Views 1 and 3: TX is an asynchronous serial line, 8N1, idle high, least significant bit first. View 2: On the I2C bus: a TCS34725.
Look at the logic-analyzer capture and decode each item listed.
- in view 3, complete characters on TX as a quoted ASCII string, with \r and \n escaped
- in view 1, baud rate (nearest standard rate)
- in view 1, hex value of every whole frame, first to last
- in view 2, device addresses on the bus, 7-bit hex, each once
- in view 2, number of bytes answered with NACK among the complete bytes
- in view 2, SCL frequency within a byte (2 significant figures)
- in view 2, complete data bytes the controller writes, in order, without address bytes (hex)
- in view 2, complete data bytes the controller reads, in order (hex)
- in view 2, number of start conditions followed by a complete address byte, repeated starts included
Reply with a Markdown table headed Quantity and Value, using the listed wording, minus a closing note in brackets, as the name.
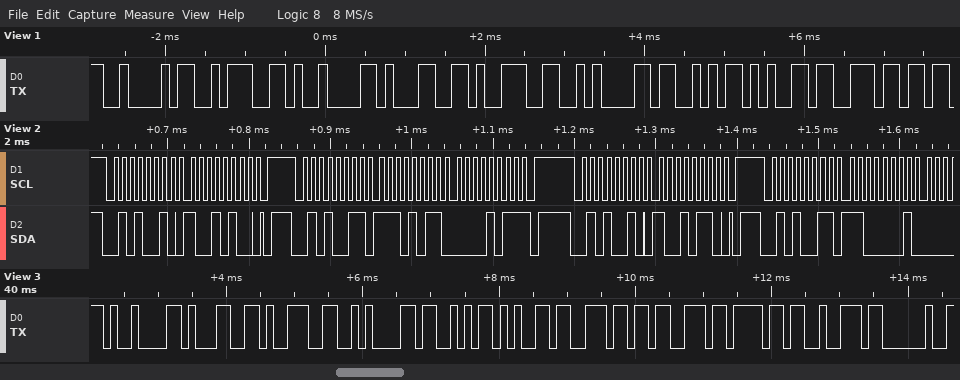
| Quantity | Value |
|---|---|
| in view 3, complete characters on TX as a quoted ASCII string, with \r and \n escaped | "\t19\nSensor " |
| in view 1, baud rate | 9600 baud |
| in view 1, hex value of every whole frame, first to last | 42 3A 09 31 39 0A 53 65 6E |
| in view 2, device addresses on the bus, 7-bit hex, each once | 0x29 |
| in view 2, number of bytes answered with NACK among the complete bytes | 1 |
| in view 2, SCL frequency within a byte | 100 kHz |
| in view 2, complete data bytes the controller writes, in order, without address bytes | 94 96 |
| in view 2, complete data bytes the controller reads, in order | EB 0B C1 |
| in view 2, number of start conditions followed by a complete address byte, repeated starts included | 4 |
